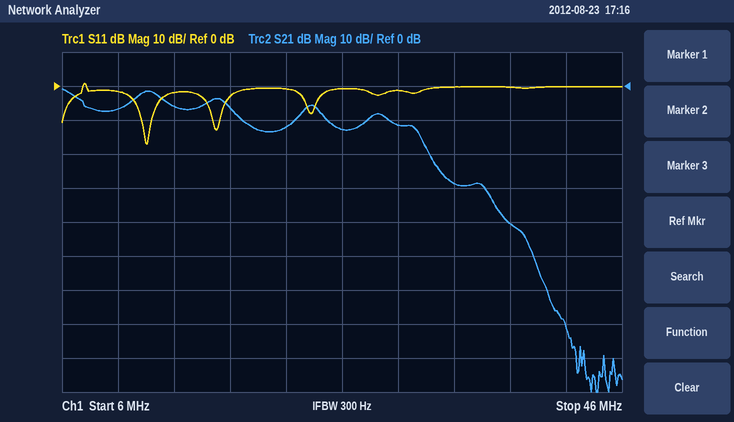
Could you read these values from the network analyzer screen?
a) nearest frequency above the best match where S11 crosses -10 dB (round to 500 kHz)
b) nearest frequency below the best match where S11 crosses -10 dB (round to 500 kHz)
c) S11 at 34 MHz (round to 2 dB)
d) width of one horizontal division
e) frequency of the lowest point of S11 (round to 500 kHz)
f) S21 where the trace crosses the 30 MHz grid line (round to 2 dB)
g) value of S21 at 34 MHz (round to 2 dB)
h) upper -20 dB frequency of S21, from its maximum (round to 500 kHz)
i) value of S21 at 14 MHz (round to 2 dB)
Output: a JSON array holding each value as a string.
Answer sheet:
["12.5 MHz", "11.5 MHz", "0 dB", "4 MHz", "12.0 MHz", "-12 dB", "-28 dB", "32.5 MHz", "-6 dB"]
